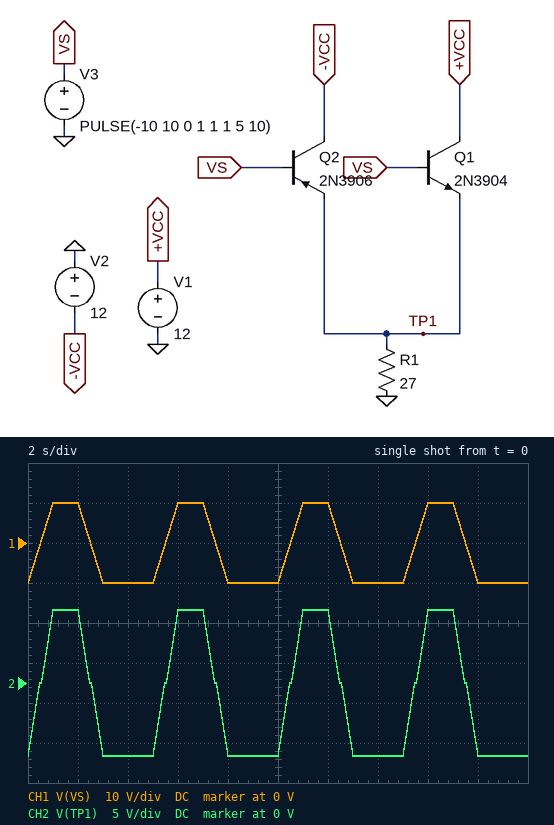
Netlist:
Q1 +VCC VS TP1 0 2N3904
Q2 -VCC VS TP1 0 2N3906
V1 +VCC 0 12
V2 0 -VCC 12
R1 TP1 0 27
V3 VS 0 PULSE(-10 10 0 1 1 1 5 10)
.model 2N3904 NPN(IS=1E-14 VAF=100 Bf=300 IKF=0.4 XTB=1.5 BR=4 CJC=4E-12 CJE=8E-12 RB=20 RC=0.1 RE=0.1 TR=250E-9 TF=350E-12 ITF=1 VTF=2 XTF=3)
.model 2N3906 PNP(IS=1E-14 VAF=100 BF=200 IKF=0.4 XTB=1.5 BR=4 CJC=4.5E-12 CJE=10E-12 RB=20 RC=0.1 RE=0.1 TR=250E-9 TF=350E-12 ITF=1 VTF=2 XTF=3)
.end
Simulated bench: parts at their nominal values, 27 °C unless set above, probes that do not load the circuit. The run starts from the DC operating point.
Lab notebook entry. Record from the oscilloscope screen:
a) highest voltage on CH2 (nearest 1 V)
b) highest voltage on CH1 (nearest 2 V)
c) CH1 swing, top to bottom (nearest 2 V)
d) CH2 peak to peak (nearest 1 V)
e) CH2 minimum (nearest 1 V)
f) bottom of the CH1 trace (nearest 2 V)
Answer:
9 V
10 V
20 V
18 V
-9 V
-10 V
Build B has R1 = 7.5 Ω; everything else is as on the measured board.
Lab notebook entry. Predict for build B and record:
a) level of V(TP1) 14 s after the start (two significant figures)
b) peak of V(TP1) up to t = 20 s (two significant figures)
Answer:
-8.6 V
8.7 V
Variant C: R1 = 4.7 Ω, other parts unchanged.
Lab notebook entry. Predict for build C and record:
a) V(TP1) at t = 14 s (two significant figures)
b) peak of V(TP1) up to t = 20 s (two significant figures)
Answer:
-8.1 V
8.3 V
